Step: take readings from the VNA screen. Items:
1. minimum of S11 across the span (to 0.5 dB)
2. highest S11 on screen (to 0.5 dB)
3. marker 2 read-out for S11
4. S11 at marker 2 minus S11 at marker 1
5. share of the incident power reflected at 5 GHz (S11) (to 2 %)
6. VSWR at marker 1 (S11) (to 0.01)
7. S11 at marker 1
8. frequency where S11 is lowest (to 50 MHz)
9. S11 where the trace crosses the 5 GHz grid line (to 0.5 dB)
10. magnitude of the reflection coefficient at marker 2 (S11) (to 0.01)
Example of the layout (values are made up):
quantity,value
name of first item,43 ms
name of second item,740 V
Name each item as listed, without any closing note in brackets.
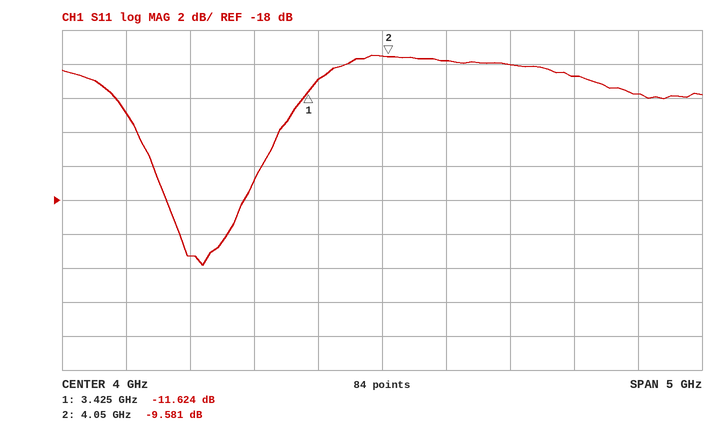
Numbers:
quantity,value
minimum of S11 across the span,-22.0 dB
highest S11 on screen,-9.5 dB
marker 2 read-out for S11,-9.581 dB
S11 at marker 2 minus S11 at marker 1,2.043 dB
share of the incident power reflected at 5 GHz (S11),10 %
VSWR at marker 1 (S11),1.71
S11 at marker 1,-11.624 dB
frequency where S11 is lowest,2.60 GHz
S11 where the trace crosses the 5 GHz grid line,-10.0 dB
magnitude of the reflection coefficient at marker 2 (S11),0.33
